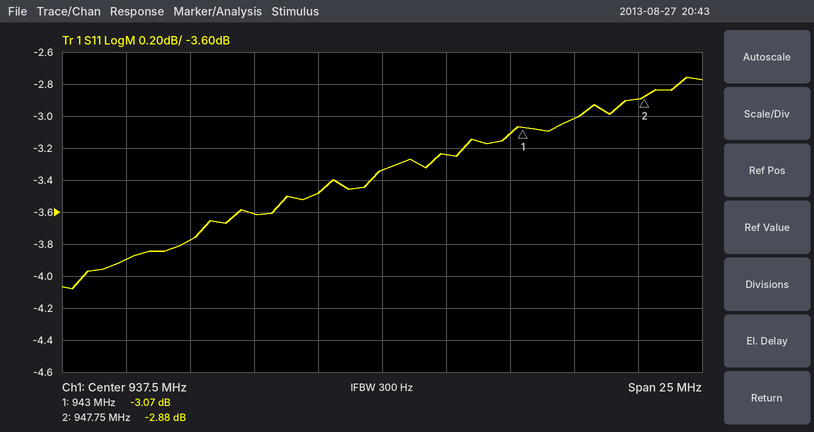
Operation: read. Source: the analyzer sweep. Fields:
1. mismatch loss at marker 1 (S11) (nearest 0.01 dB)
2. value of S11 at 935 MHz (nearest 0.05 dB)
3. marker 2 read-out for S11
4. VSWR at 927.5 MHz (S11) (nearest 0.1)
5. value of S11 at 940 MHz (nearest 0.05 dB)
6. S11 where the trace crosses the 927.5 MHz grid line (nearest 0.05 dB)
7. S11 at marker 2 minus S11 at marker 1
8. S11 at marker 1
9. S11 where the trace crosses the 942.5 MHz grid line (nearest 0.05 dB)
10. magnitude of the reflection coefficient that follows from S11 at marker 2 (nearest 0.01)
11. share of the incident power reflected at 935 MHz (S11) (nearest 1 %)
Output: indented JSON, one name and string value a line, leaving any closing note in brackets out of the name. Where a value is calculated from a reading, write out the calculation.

{
  "mismatch loss at marker 1 (S11)": "−10 log10(1 − 10^(-3.07/10)) ≈ 2.95 dB",
  "value of S11 at 935 MHz": "-3.50 dB",
  "marker 2 read-out for S11": "-2.88 dB",
  "VSWR at 927.5 MHz (S11)": "|Γ| = 10^(-3.9/20) = 0.6383; VSWR = (1 + 0.6383)/(1 − 0.6383) ≈ 4.5",
  "value of S11 at 940 MHz": "-3.25 dB",
  "S11 where the trace crosses the 927.5 MHz grid line": "-3.90 dB",
  "S11 at marker 2 minus S11 at marker 1": "-2.88 − (-3.07) = 0.19 dB",
  "S11 at marker 1": "-3.07 dB",
  "S11 where the trace crosses the 942.5 MHz grid line": "-3.10 dB",
  "magnitude of the reflection coefficient that follows from S11 at marker 2": "10^(-2.88/20) ≈ 0.72",
  "share of the incident power reflected at 935 MHz (S11)": "10^(-3.5/10) ≈ 45 %"
}
